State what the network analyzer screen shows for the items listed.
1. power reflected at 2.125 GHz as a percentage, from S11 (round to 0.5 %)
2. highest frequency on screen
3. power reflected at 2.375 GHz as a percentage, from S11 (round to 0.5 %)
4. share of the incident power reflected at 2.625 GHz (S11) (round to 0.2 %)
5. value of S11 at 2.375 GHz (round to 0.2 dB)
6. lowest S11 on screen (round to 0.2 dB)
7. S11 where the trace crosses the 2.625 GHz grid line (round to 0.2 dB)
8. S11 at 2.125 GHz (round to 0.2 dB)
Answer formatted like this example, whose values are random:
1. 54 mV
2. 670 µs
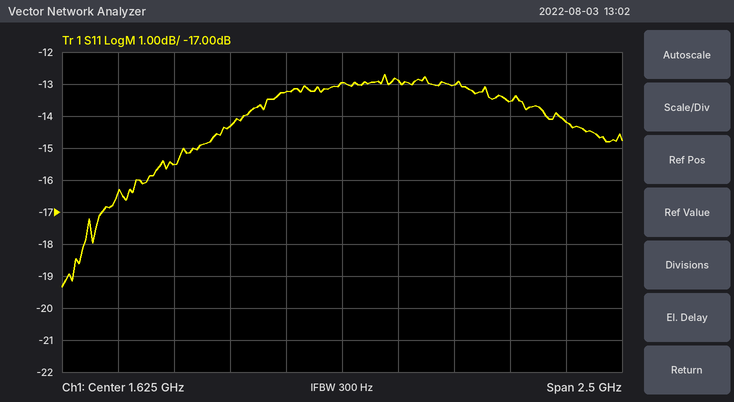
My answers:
1. 5.0 %
2. 2.875 GHz
3. 4.5 %
4. 3.8 %
5. -13.6 dB
6. -19.4 dB
7. -14.2 dB
8. -13.0 dB
